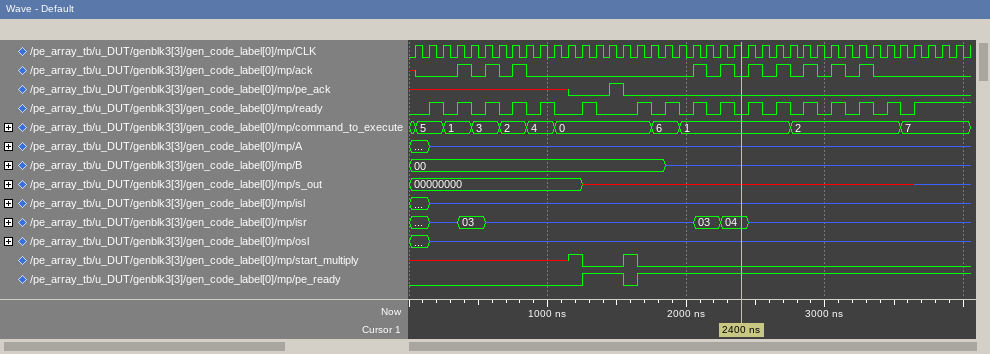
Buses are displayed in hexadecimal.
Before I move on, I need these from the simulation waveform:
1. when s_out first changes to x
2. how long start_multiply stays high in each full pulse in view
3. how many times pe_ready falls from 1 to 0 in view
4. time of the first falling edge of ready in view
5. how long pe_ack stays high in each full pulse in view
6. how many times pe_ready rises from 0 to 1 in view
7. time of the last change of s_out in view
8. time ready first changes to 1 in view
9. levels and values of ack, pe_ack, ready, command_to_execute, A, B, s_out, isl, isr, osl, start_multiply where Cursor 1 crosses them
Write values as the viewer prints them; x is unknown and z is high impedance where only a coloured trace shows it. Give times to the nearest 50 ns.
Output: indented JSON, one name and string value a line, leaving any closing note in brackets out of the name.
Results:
{
  "when s_out first changes to x": "1250 ns",
  "how long start_multiply stays high in each full pulse in view": "100 ns",
  "how many times pe_ready falls from 1 to 0 in view": "1",
  "time of the first falling edge of ready in view": "250 ns",
  "how long pe_ack stays high in each full pulse in view": "100 ns",
  "how many times pe_ready rises from 0 to 1 in view": "2",
  "time of the last change of s_out in view": "3650 ns",
  "time ready first changes to 1 in view": "150 ns",
  "levels and values of ack, pe_ack, ready, command_to_execute, A, B, s_out, isl, isr, osl, start_multiply where Cursor 1 crosses them": "ack=0, pe_ack=0, ready=0, command_to_execute=1, A=z, B=z, s_out=x, isl=z, isr=04, osl=z, start_multiply=0"
}
